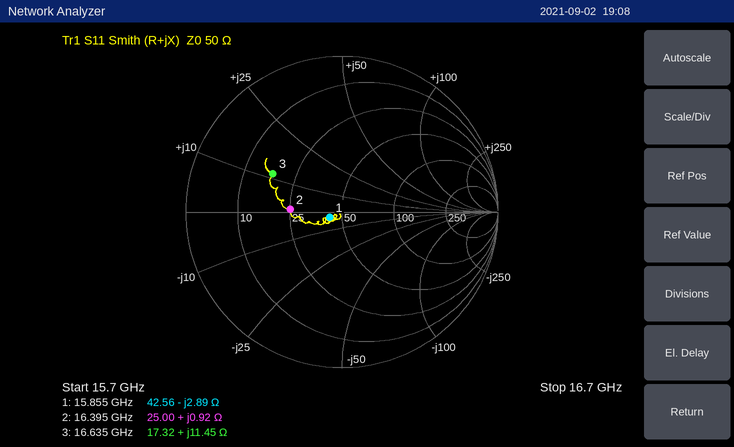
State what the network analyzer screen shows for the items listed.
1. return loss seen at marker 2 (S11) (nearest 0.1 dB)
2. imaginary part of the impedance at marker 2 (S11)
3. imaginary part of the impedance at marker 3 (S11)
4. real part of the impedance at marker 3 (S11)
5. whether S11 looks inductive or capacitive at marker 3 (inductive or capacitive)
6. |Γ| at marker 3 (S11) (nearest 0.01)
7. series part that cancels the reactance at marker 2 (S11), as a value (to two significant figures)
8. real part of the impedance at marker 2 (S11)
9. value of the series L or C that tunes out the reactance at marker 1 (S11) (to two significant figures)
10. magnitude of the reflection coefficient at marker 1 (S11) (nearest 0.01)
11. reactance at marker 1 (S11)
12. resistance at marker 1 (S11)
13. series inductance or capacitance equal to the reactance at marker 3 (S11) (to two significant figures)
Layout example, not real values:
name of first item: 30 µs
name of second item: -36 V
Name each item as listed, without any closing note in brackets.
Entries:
return loss seen at marker 2 (S11): 9.5 dB
imaginary part of the impedance at marker 2: +0.92 Ω
imaginary part of the impedance at marker 3: +11.45 Ω
real part of the impedance at marker 3: 17.32 Ω
whether S11 looks inductive or capacitive at marker 3: inductive
|Γ| at marker 3 (S11): 0.51
series part that cancels the reactance at marker 2 (S11), as a value: 11 pF
real part of the impedance at marker 2: 25.00 Ω
value of the series L or C that tunes out the reactance at marker 1 (S11): 29 pH
magnitude of the reflection coefficient at marker 1 (S11): 0.09
reactance at marker 1: -2.89 Ω
resistance at marker 1: 42.56 Ω
series inductance or capacitance equal to the reactance at marker 3 (S11): 110 pH
